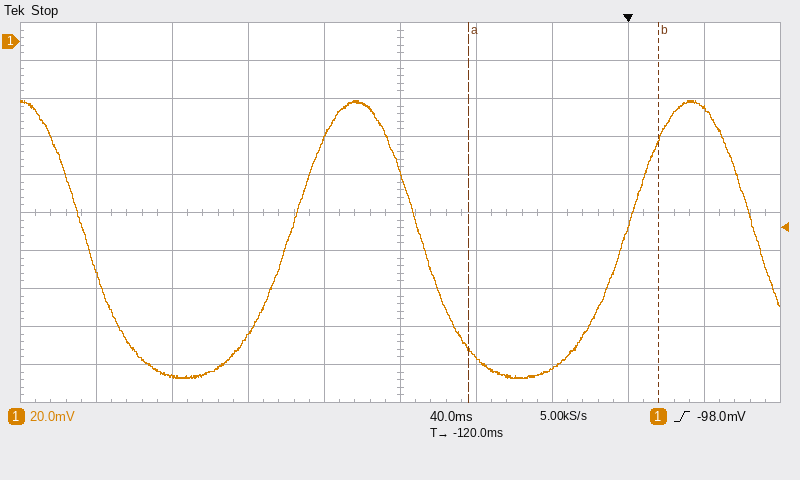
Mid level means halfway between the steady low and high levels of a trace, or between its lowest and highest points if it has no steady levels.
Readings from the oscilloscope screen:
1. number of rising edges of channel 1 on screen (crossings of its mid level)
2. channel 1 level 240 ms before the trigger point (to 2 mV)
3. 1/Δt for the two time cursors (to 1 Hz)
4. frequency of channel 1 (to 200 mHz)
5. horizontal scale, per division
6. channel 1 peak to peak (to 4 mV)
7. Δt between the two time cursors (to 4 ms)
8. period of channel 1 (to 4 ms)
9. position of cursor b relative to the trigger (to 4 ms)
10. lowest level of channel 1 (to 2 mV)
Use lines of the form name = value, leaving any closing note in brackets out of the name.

number of rising edges of channel 1 on screen = 2
channel 1 level 240 ms before the trigger point = -176 mV
1/Δt for the two time cursors = 10 Hz
frequency of channel 1 = 5.6 Hz
horizontal scale, per division = 40 ms
channel 1 peak to peak = 148 mV
Δt between the two time cursors = 100 ms
period of channel 1 = 176 ms
position of cursor b relative to the trigger = +16 ms
lowest level of channel 1 = -178 mV
